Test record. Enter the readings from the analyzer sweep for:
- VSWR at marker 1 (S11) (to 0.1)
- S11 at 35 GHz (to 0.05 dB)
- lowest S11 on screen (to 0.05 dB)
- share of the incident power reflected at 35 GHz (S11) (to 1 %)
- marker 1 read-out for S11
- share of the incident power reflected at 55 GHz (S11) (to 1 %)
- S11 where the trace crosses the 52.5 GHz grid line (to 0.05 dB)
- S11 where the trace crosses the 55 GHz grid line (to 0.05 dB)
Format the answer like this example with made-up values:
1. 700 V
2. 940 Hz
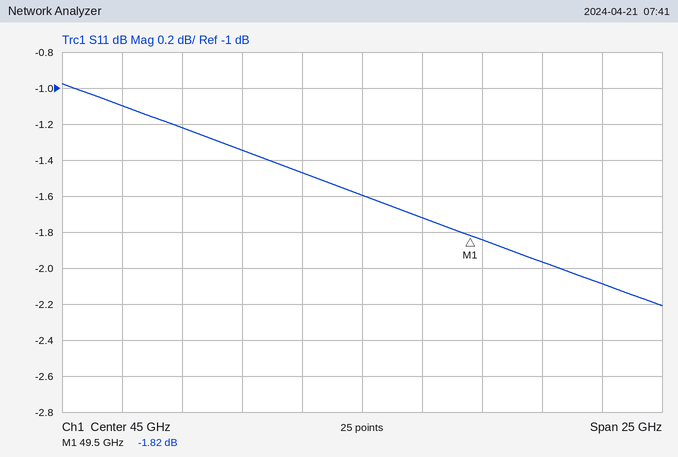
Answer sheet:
1. 9.6
2. -1.10 dB
3. -2.20 dB
4. 78 %
5. -1.82 dB
6. 62 %
7. -1.95 dB
8. -2.10 dB
